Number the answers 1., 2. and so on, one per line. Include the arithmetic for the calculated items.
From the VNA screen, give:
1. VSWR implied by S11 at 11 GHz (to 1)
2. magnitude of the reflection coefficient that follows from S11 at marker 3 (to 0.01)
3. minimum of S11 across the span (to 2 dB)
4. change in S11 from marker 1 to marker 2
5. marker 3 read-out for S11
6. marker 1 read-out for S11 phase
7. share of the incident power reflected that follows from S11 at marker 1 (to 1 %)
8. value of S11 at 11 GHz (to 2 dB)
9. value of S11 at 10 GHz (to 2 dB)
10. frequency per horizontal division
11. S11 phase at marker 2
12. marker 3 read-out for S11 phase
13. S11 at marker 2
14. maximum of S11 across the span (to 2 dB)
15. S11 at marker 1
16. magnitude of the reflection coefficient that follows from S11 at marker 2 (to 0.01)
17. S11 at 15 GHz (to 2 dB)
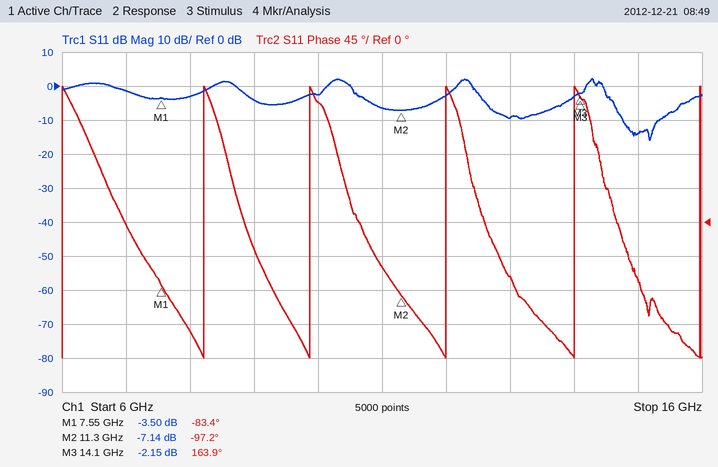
1. |Γ| = 10^(-6/20) = 0.5012; VSWR = (1 + 0.5012)/(1 − 0.5012) ≈ 3
2. 10^(-2.15/20) ≈ 0.78
3. -16 dB
4. -7.14 − (-3.5) = -3.64 dB
5. -2.15 dB
6. -83.4°
7. 10^(-3.5/10) ≈ 45 %
8. -6 dB
9. -2 dB
10. 1 GHz
11. -97.2°
12. 163.9°
13. -7.14 dB
14. 2 dB
15. -3.50 dB
16. 10^(-7.14/20) ≈ 0.44
17. -14 dB
